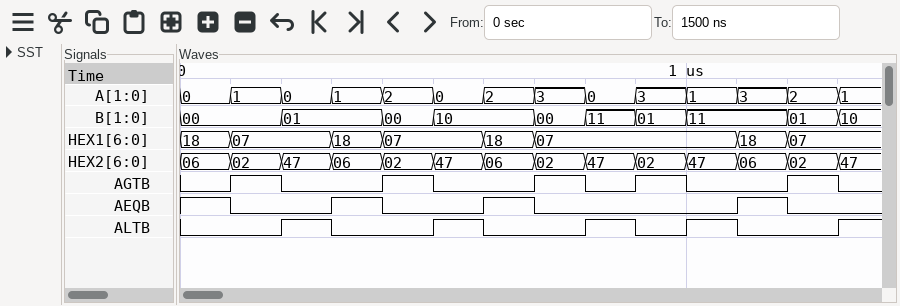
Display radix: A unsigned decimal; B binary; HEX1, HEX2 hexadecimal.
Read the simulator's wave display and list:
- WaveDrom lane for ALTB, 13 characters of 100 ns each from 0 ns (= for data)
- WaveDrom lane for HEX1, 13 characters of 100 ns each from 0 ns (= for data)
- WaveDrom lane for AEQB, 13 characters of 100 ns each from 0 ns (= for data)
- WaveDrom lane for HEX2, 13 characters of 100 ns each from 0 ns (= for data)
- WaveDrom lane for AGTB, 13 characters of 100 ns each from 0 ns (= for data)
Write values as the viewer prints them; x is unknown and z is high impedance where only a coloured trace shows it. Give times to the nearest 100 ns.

{name: 'ALTB', wave: '0.10.10.1010.'}
{name: 'HEX1', wave: '==.==.==...==', data: '18 07 18 07 18 07 18 07'}
{name: 'AEQB', wave: '10.10.10...10'}
{name: 'HEX2', wave: '=============', data: '06 02 47 06 02 47 06 02 47 02 47 06 02'}
{name: 'AGTB', wave: '010.10.1010.1'}
